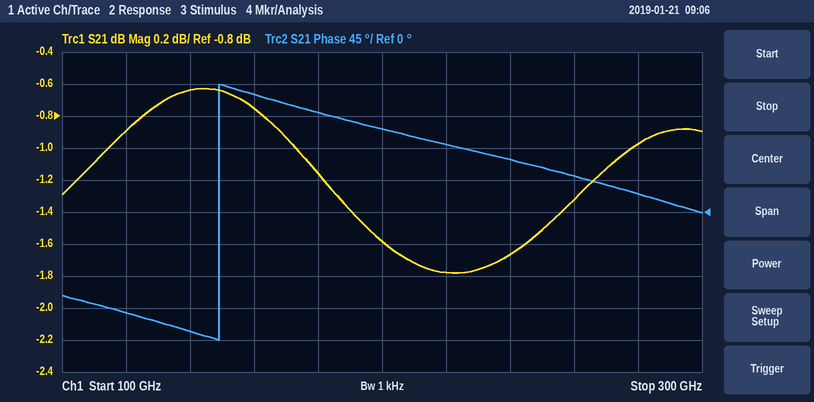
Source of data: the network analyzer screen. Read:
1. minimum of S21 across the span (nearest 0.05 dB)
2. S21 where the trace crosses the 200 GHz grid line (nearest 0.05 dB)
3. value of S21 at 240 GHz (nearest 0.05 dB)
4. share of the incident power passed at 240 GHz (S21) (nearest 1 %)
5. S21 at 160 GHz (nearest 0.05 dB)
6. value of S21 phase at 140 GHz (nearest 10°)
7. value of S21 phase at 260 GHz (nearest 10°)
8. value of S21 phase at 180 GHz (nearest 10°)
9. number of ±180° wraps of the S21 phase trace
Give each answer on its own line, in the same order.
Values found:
-1.80 dB
-1.60 dB
-1.65 dB
68 %
-0.75 dB
-170°
50°
140°
1
